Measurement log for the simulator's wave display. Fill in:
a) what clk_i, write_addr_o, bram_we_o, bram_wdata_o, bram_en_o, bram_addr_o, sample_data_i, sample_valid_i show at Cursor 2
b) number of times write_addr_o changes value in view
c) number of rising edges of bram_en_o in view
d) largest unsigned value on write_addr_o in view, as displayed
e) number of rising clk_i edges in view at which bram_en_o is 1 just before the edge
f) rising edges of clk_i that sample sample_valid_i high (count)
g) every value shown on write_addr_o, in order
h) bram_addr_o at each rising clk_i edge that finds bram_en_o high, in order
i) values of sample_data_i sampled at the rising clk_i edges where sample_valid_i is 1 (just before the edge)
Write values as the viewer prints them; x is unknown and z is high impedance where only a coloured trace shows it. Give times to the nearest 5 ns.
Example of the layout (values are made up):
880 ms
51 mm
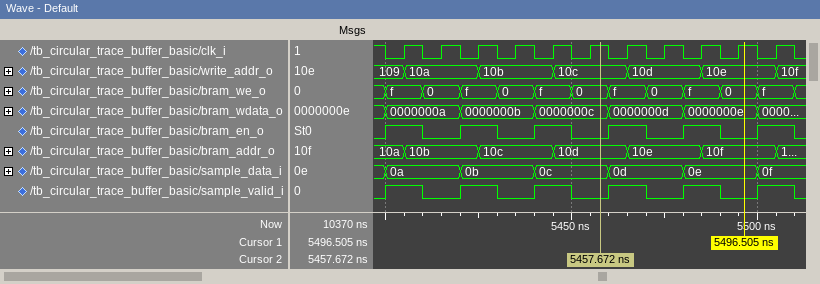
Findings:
clk_i=1, write_addr_o=10c, bram_we_o=0, bram_wdata_o=0000000c, bram_en_o=0, bram_addr_o=10d, sample_data_i=0c, sample_valid_i=0
6
6
10f
6
6
109, 10a, 10b, 10c, 10d, 10e, 10f
10a, 10b, 10c, 10d, 10e, 10f
0a, 0b, 0c, 0d, 0e, 0f
